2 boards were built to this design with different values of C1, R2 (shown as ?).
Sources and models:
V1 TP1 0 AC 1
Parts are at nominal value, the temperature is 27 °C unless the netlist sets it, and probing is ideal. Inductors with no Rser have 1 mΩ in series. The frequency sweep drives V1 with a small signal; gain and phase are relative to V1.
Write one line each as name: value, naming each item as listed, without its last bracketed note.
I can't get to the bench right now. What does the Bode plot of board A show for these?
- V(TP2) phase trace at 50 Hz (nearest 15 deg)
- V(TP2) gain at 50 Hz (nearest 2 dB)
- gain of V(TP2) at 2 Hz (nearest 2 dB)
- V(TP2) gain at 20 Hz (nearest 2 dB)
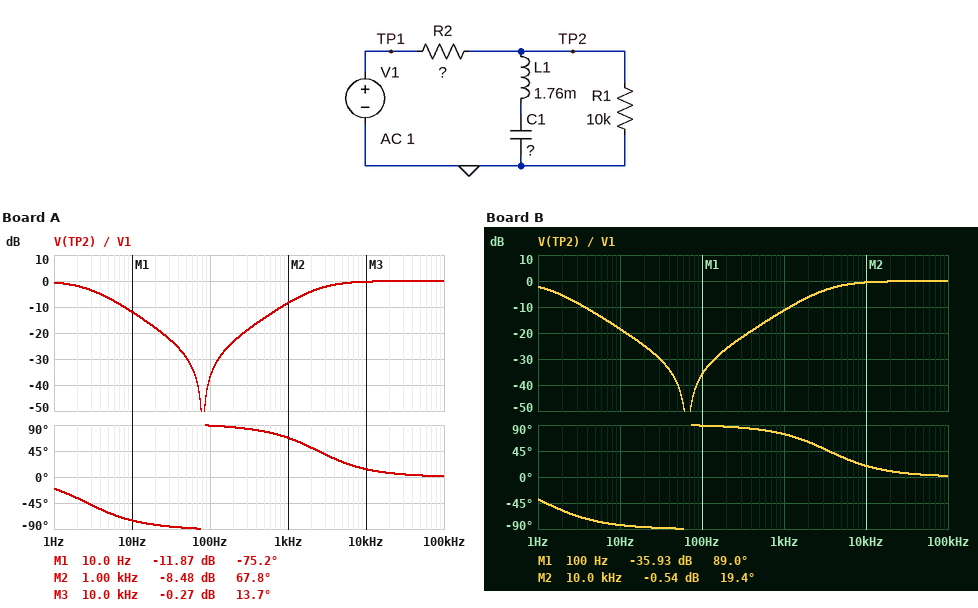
V(TP2) phase trace at 50 Hz: -90 deg
V(TP2) gain at 50 Hz: -30 dB
gain of V(TP2) at 2 Hz: -2 dB
V(TP2) gain at 20 Hz: -18 dB
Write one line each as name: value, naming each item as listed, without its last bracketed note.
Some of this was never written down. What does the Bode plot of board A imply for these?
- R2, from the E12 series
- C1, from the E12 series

R2, from the E12 series: 27 Ω
C1, from the E12 series: 2.2 mF
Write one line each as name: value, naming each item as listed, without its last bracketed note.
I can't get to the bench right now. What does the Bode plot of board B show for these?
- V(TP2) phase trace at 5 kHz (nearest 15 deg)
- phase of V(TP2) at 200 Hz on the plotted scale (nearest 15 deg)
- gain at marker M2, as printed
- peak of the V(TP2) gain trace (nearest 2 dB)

V(TP2) phase trace at 5 kHz: 30 deg
phase of V(TP2) at 200 Hz on the plotted scale: 90 deg
gain at marker M2, as printed: -0.54 dB
peak of the V(TP2) gain trace: 0 dB
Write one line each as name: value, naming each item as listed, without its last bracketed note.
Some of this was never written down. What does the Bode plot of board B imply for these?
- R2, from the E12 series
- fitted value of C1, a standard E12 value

R2, from the E12 series: 39 Ω
fitted value of C1, a standard E12 value: 3.3 mF
